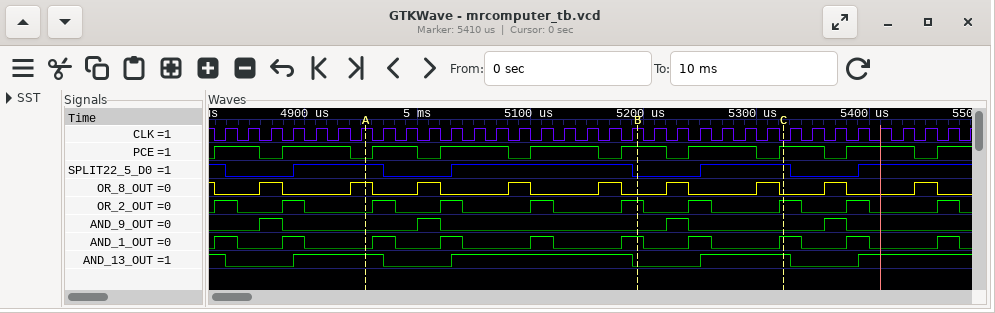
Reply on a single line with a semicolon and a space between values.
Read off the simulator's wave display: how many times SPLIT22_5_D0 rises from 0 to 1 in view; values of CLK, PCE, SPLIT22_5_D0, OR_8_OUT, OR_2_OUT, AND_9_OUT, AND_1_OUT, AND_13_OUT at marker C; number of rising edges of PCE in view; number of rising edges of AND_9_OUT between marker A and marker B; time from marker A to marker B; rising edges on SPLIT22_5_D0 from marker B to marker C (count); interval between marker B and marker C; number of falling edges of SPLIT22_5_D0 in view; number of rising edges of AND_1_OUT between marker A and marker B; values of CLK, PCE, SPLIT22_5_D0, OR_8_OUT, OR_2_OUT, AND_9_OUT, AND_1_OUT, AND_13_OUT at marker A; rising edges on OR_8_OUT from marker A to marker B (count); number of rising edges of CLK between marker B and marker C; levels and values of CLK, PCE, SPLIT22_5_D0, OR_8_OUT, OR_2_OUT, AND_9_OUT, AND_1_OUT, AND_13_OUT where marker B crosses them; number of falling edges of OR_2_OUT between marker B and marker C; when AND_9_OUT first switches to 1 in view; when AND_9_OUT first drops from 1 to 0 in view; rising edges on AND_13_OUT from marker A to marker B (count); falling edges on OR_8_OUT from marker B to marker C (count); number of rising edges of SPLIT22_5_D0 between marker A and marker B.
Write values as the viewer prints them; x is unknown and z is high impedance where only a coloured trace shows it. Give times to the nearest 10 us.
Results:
4; CLK=0, PCE=1, SPLIT22_5_D0=1, OR_8_OUT=0, OR_2_OUT=1, AND_9_OUT=0, AND_1_OUT=1, AND_13_OUT=1; 10; 1; 240 us; 1; 130 us; 4; 4; CLK=1, PCE=0, SPLIT22_5_D0=1, OR_8_OUT=1, OR_2_OUT=0, AND_9_OUT=0, AND_1_OUT=0, AND_13_OUT=1; 3; 6; CLK=1, PCE=1, SPLIT22_5_D0=0, OR_8_OUT=0, OR_2_OUT=1, AND_9_OUT=0, AND_1_OUT=1, AND_13_OUT=0; 2; 4860 us; 4880 us; 1; 2; 1
